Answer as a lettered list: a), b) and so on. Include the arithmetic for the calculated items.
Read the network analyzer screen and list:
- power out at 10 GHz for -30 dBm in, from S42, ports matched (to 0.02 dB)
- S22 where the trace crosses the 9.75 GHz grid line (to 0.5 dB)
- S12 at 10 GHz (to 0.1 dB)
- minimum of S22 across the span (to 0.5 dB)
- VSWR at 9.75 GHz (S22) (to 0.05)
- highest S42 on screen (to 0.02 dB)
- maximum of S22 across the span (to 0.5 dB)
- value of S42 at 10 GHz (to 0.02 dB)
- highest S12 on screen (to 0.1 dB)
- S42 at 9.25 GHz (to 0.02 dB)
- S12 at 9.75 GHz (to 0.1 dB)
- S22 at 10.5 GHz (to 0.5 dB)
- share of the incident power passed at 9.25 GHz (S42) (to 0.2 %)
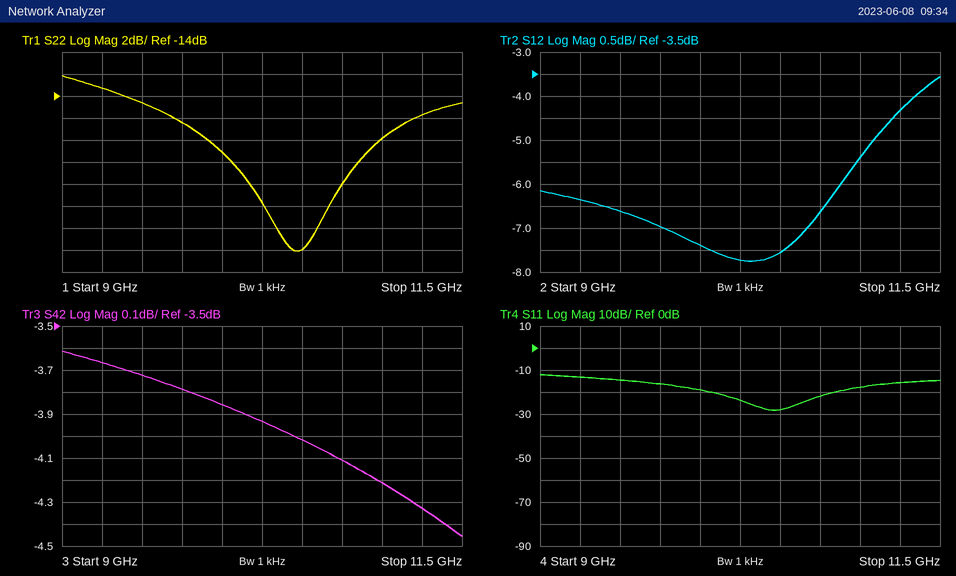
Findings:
a) -30 dBm + (-3.86 dB) = -33.86 dBm
b) -16.5 dB
c) -7.4 dB
d) -28.0 dB
e) |Γ| = 10^(-16.5/20) = 0.1496; VSWR = (1 + 0.1496)/(1 − 0.1496) ≈ 1.35
f) -3.62 dB
g) -12.0 dB
h) -3.86 dB
i) -3.6 dB
j) -3.66 dB
k) -7.0 dB
l) -28.0 dB
m) 10^(-3.66/10) ≈ 43.1 %, so 43.0 % to the nearest 0.2 %
